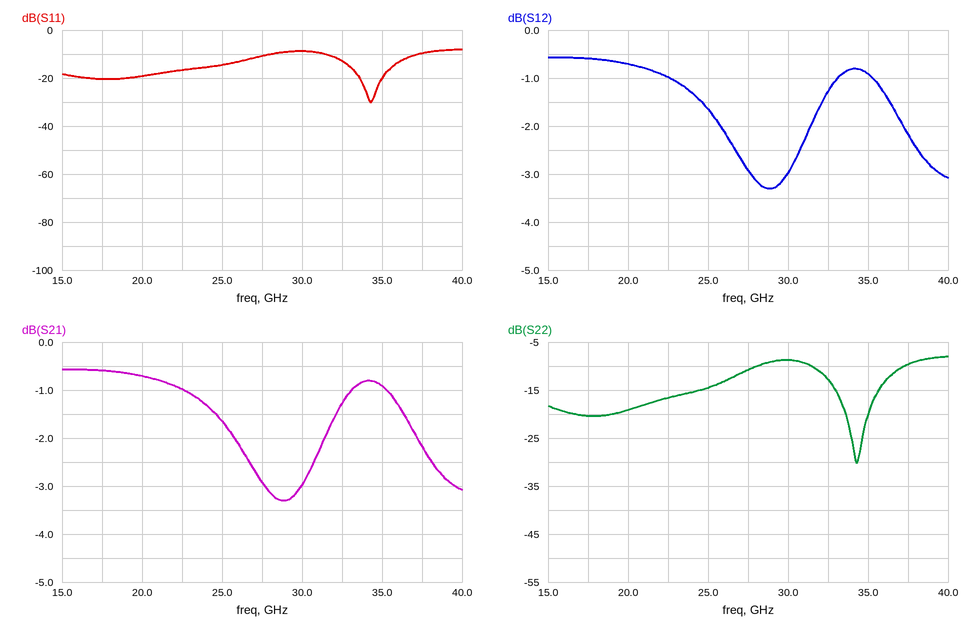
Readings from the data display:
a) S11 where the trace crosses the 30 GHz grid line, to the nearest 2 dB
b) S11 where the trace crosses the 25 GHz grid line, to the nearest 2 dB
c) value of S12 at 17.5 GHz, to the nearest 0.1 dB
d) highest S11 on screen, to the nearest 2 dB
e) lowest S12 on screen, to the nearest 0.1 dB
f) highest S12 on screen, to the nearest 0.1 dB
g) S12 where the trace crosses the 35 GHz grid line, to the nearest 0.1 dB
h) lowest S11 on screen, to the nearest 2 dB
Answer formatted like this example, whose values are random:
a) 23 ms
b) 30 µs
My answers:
a) -8 dB
b) -14 dB
c) -0.6 dB
d) -8 dB
e) -3.3 dB
f) -0.6 dB
g) -0.9 dB
h) -30 dB
